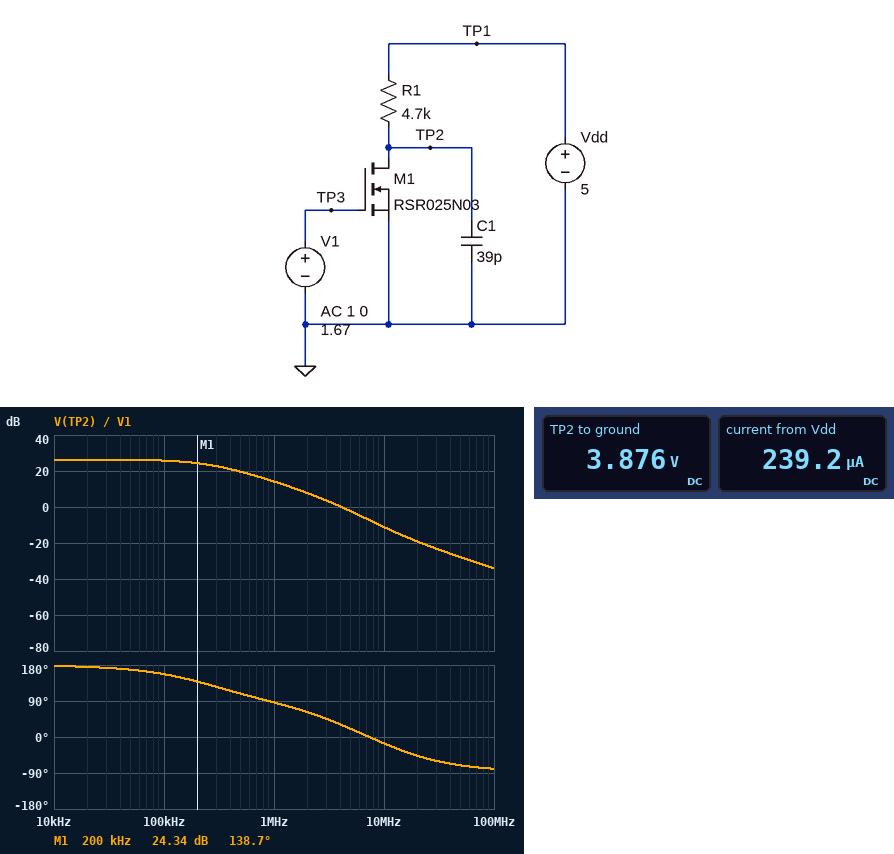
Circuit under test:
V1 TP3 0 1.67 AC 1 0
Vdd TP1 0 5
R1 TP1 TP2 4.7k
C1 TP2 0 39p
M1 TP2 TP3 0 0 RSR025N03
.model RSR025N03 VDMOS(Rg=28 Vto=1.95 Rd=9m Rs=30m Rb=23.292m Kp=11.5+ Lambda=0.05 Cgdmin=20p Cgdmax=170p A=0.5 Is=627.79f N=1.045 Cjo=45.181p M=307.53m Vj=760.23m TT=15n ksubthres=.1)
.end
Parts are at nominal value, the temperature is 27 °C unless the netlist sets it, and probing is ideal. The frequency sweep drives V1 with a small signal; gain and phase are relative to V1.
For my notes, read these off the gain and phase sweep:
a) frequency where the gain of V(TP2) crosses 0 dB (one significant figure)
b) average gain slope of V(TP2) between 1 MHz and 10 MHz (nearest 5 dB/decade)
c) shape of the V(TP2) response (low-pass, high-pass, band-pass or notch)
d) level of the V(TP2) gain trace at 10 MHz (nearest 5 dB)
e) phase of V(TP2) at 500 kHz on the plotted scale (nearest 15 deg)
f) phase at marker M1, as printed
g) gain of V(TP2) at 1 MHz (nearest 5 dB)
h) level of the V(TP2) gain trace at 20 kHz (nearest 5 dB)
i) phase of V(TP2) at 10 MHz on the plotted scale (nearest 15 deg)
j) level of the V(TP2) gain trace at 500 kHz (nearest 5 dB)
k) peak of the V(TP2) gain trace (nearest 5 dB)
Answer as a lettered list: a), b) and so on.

a) 4 MHz
b) -25 dB/decade
c) low-pass
d) -10 dB
e) 105 deg
f) 138.7 deg
g) 15 dB
h) 25 dB
i) -15 deg
j) 20 dB
k) 25 dB
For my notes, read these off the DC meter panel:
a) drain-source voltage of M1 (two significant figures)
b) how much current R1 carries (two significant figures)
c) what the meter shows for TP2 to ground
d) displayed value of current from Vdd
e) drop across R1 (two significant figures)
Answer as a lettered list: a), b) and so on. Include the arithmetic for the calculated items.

a) 3.876 V = 3.9 V
b) (5 V - 3.876 V) / 4.7 kΩ = 240 µA
c) 3.876 V
d) 239.2 µA
e) 5 V - 3.876 V = 1.1 V
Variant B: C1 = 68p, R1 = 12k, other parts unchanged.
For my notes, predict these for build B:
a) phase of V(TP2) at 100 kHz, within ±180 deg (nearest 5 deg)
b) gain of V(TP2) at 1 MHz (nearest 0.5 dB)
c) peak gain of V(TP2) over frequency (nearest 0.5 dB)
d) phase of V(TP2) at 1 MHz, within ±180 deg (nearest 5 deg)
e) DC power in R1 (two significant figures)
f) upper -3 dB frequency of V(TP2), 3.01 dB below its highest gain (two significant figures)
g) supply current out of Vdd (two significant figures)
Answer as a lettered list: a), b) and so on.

a) 125 deg
b) 10.5 dB
c) 33.5 dB
d) 75 deg
e) 600 µW
f) 73 kHz
g) 220 µA
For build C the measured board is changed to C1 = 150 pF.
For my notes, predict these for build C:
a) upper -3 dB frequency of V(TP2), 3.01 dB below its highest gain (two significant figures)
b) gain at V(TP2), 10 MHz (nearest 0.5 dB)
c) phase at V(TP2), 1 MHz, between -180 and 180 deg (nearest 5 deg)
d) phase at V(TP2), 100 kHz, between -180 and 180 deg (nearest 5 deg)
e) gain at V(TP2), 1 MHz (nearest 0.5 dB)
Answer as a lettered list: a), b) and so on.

a) 140 kHz
b) -16.5 dB
c) 80 deg
d) 145 deg
e) 9.0 dB
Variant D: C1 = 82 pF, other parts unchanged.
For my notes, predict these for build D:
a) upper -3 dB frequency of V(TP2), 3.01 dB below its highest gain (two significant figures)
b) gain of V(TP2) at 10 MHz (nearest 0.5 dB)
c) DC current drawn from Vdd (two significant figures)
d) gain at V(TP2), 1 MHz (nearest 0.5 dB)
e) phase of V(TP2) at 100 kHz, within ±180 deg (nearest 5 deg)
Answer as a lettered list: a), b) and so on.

a) 200 kHz
b) -13.5 dB
c) 240 µA
d) 12.0 dB
e) 150 deg
